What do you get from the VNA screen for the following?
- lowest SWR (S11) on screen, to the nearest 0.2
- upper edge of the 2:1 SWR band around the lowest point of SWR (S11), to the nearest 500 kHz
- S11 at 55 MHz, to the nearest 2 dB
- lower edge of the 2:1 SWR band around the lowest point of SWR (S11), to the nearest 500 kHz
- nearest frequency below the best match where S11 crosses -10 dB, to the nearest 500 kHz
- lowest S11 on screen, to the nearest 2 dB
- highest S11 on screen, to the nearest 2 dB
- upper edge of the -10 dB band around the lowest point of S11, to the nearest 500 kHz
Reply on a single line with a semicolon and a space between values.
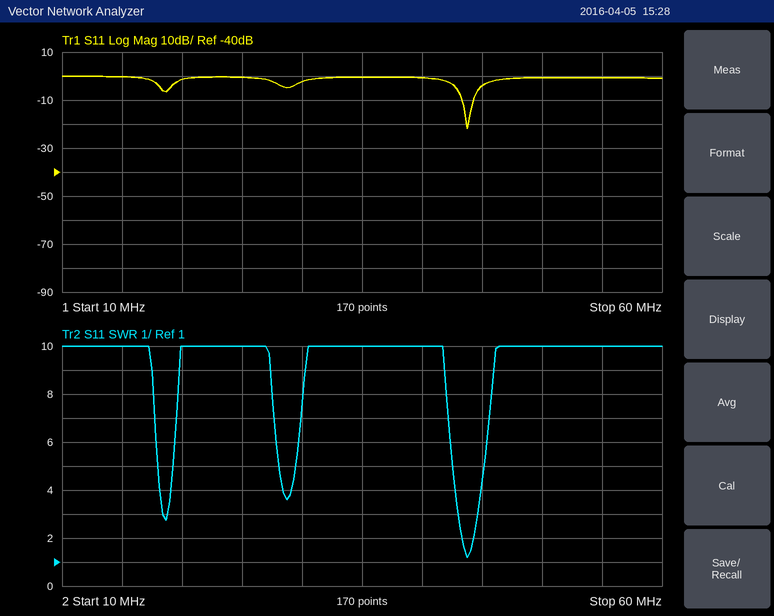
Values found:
1.2; 44.5 MHz; 0 dB; 43.5 MHz; 43.5 MHz; -22 dB; 0 dB; 44.5 MHz
